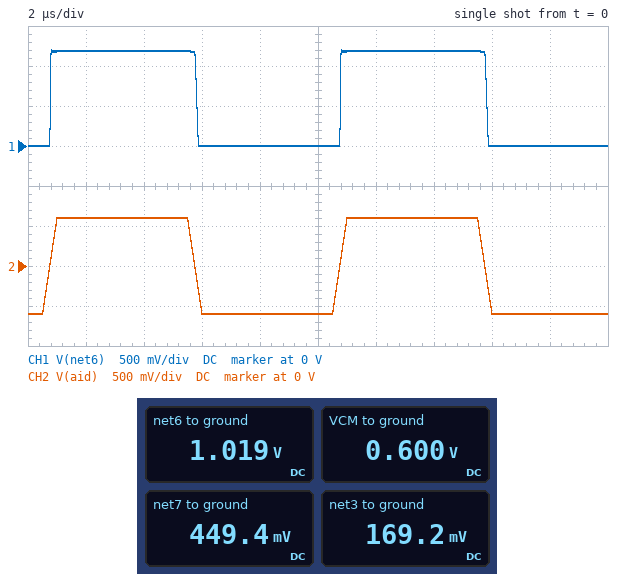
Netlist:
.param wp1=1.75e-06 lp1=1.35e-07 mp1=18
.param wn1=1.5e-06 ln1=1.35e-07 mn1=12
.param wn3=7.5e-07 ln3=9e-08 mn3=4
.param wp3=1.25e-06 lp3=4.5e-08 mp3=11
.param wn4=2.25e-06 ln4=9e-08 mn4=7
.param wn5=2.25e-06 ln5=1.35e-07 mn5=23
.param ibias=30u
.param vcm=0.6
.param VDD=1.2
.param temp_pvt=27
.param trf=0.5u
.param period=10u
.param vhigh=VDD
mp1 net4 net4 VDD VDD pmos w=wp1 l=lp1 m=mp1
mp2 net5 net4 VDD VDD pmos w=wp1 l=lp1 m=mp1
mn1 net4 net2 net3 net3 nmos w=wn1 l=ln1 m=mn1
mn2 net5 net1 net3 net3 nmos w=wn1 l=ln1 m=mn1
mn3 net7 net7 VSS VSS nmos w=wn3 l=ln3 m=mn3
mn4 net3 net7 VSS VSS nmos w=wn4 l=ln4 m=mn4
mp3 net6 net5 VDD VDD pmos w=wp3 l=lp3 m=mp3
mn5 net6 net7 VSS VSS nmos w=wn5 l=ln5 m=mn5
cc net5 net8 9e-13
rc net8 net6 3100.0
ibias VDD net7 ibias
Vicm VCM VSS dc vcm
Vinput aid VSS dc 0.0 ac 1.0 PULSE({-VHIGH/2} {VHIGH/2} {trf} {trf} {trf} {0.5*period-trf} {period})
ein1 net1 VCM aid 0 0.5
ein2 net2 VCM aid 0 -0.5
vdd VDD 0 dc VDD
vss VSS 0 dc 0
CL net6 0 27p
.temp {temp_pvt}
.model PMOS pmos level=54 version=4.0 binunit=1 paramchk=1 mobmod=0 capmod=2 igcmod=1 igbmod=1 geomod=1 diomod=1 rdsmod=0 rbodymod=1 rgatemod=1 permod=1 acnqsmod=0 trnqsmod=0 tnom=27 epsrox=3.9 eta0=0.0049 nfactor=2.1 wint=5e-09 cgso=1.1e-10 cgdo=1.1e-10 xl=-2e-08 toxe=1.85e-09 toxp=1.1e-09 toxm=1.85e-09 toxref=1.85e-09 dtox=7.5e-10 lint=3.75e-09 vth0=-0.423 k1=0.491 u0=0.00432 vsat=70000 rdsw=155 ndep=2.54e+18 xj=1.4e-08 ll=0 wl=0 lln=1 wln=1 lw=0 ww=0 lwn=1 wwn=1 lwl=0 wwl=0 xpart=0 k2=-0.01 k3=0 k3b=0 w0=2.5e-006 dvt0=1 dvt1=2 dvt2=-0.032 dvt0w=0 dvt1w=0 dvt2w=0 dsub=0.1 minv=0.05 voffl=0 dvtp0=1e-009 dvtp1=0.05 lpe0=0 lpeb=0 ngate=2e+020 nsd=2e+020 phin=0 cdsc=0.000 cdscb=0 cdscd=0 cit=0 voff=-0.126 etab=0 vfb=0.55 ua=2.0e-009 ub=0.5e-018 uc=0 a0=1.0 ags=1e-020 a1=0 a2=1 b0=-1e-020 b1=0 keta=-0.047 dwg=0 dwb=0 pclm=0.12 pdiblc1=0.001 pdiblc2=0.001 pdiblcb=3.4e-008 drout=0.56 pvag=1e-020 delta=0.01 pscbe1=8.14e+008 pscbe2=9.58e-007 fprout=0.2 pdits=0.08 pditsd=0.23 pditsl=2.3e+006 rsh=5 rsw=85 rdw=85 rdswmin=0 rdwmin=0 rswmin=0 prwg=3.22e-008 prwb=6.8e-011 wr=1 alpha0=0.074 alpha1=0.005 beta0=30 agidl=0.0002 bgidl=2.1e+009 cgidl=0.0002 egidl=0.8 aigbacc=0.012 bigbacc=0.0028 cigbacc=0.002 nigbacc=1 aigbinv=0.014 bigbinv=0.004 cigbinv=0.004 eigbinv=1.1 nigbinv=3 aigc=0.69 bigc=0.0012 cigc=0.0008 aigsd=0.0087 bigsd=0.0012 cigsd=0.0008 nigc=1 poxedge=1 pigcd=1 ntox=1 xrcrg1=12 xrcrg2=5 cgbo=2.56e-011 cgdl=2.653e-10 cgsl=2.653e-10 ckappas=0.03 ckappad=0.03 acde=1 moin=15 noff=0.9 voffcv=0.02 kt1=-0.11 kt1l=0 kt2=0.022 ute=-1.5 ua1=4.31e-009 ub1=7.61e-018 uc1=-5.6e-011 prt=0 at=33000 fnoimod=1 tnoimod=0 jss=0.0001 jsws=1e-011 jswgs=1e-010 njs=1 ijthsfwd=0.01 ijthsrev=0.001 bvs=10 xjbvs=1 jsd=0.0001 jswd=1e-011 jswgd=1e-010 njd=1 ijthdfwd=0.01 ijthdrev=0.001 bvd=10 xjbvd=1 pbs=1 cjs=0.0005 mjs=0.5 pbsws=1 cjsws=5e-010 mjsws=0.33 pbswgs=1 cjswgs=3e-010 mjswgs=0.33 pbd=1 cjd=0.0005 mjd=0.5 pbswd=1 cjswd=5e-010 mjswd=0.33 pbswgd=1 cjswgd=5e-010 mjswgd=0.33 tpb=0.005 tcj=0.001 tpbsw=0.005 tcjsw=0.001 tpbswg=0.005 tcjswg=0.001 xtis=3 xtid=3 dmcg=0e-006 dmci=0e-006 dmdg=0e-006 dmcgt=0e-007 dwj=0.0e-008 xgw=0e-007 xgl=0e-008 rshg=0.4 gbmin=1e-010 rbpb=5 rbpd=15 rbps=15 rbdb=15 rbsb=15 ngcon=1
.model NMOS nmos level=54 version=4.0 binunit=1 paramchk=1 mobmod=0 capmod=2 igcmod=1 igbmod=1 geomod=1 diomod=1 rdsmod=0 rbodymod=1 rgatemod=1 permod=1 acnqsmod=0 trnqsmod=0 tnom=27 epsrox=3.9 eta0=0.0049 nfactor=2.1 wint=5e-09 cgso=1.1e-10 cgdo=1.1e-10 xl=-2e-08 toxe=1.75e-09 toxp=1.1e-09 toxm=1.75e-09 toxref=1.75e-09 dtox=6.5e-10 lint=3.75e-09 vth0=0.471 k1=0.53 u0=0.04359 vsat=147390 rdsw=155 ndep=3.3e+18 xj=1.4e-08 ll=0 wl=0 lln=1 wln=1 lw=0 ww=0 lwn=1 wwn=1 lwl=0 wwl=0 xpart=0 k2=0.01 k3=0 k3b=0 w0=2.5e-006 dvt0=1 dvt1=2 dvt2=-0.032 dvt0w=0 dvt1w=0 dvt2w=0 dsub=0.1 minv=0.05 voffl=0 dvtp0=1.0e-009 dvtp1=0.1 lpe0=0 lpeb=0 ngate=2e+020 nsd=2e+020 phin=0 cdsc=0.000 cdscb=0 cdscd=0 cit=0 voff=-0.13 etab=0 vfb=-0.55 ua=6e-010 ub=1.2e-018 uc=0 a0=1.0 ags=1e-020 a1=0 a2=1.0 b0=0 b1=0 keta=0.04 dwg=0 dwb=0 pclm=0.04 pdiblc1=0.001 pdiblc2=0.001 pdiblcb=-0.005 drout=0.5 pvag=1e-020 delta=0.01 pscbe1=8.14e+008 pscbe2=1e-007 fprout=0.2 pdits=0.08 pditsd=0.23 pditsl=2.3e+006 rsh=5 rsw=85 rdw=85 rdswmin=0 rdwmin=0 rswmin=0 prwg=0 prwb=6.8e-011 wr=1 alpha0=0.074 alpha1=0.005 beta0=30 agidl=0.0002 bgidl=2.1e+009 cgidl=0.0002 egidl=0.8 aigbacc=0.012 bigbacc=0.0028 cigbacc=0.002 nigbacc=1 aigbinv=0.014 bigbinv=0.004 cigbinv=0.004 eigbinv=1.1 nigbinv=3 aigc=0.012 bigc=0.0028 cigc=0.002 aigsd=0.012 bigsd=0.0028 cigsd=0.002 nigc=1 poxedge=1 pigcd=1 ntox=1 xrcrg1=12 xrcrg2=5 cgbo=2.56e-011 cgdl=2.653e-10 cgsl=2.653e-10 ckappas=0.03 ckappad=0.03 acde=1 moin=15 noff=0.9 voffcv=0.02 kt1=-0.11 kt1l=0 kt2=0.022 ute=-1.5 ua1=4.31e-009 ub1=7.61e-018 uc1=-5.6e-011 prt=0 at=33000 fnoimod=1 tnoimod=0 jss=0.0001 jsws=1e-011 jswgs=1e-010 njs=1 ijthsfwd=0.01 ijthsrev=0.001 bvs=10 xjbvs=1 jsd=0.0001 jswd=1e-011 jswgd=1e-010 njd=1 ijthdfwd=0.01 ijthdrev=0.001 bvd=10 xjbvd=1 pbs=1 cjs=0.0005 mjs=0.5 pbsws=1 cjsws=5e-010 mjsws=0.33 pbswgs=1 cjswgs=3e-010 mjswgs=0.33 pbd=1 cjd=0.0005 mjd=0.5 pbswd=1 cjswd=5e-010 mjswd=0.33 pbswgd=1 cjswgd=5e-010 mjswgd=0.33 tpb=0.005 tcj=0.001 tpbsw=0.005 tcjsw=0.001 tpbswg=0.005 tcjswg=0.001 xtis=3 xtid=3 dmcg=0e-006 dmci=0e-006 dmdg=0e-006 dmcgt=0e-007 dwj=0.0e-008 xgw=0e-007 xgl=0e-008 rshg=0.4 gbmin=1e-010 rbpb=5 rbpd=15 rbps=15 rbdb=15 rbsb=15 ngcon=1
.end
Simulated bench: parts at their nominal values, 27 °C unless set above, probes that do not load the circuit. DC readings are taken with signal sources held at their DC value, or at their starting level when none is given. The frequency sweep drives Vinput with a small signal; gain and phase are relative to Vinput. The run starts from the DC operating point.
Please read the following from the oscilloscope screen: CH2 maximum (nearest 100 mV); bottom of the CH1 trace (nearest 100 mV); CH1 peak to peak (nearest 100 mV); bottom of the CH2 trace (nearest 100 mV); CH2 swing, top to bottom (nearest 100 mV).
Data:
600 mV
0 V
1.2 V
-600 mV
1.2 V
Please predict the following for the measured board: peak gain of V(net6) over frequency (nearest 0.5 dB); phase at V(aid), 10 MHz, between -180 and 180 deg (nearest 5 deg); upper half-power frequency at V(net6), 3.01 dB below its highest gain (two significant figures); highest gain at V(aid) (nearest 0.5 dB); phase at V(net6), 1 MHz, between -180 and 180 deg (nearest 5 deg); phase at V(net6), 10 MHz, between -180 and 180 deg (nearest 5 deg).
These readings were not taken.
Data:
46.5 dB
0 deg
740 kHz
0 dB
-55 deg
-100 deg
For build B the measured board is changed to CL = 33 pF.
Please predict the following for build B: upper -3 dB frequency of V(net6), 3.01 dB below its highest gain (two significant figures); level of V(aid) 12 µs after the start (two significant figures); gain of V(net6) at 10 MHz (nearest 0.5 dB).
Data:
730 kHz
600 mV
23.0 dB
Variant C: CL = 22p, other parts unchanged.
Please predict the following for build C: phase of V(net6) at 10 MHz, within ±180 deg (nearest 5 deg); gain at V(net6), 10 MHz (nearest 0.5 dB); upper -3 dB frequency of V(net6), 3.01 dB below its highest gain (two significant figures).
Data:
-95 deg
24.0 dB
760 kHz
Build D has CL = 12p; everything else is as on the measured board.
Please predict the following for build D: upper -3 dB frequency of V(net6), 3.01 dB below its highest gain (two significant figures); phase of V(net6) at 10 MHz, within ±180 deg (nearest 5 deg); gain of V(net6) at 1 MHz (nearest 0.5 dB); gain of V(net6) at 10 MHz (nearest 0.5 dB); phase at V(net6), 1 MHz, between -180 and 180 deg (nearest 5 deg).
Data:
780 kHz
-85 deg
42.5 dB
24.5 dB
-50 deg
